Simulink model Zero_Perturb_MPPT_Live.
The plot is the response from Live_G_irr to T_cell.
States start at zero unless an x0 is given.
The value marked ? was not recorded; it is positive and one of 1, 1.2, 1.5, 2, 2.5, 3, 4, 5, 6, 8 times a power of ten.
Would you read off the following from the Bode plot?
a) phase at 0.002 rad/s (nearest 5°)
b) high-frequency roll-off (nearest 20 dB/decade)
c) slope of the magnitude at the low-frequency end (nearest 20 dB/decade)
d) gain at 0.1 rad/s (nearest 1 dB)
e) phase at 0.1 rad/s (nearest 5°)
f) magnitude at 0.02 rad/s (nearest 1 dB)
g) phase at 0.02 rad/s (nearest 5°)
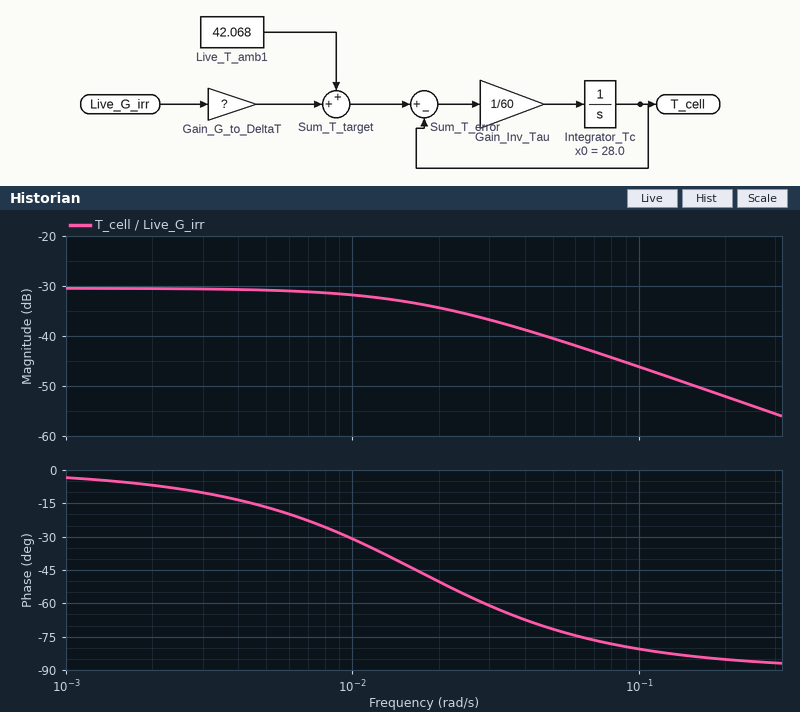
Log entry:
-5°
-20 dB/decade
0 dB/decade
-46 dB
-80°
-34 dB
-50°
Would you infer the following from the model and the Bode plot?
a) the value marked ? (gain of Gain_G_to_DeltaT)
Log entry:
0.03
